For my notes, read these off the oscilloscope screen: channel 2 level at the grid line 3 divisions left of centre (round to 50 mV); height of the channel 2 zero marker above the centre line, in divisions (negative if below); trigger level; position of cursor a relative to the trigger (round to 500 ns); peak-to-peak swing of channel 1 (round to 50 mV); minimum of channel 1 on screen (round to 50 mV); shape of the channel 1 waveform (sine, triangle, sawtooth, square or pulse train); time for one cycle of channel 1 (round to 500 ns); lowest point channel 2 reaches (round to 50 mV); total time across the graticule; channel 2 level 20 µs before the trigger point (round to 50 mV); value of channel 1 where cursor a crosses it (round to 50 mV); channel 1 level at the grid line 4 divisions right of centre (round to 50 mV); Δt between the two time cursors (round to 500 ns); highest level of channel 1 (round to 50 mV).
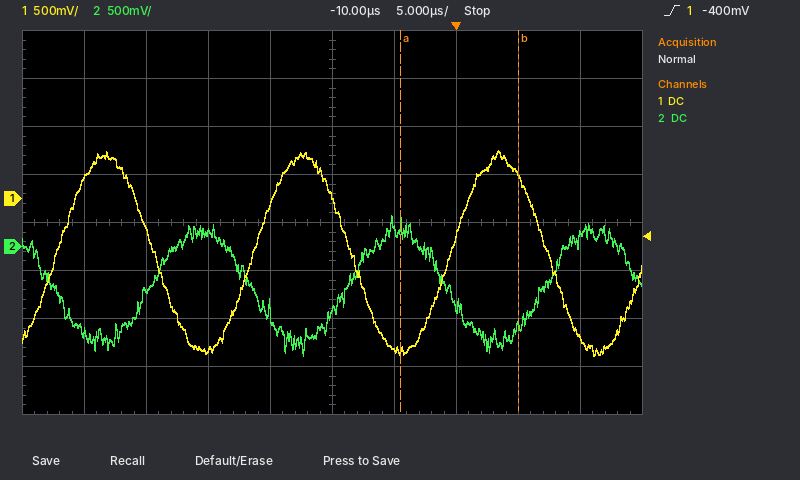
-450 mV
-0.5 div
-400 mV
-4.5 µs
2.15 V
-1.65 V
sine
16.0 µs
-1.15 V
50 µs
150 mV
-1.60 V
-1.45 V
9.5 µs
500 mV
